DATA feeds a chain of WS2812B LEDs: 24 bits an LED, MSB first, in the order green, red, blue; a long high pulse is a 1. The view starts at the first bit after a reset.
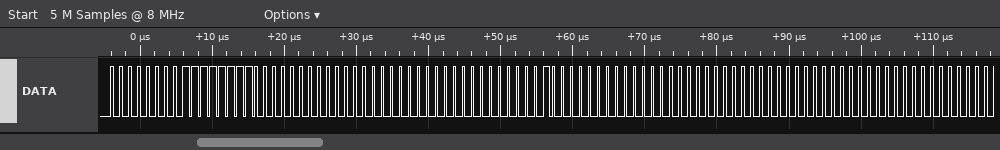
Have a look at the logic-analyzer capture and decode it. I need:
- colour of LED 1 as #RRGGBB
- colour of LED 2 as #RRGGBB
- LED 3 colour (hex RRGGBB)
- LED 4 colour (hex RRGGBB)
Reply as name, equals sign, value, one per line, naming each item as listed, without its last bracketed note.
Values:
colour of LED 1 as #RRGGBB = #FF0000
colour of LED 2 as #RRGGBB = #000000
LED 3 colour = #008000
LED 4 colour = #000000
